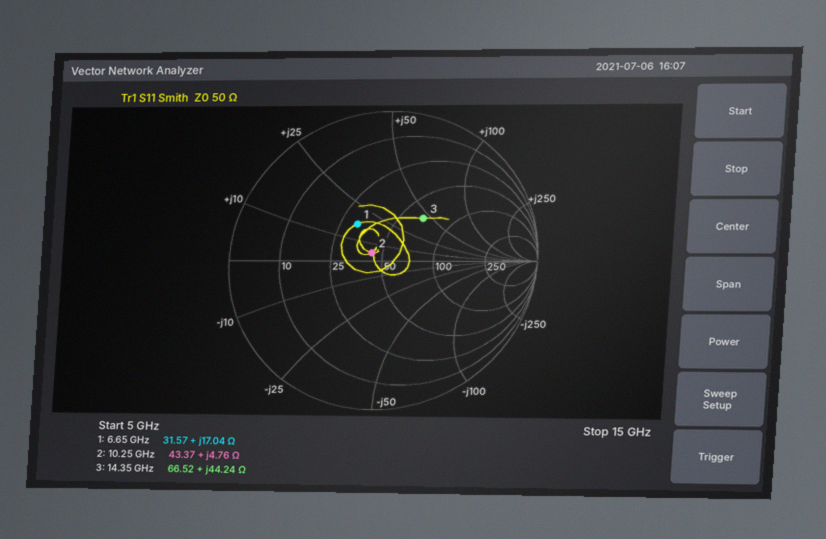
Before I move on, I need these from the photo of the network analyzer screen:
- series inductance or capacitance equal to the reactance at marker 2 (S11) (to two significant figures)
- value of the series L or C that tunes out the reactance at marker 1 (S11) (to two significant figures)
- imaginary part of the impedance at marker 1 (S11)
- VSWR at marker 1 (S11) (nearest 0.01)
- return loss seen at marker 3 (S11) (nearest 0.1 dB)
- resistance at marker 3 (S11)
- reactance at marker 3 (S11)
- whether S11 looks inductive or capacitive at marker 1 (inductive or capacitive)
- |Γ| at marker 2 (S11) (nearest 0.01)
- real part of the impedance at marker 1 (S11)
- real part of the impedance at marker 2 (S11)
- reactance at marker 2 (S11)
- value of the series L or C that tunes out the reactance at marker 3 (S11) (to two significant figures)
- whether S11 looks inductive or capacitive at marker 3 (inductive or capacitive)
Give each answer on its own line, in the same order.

74 pH
1.4 pF
+17.04 Ω
1.86
8.4 dB
66.52 Ω
+44.24 Ω
inductive
0.09
31.57 Ω
43.37 Ω
+4.76 Ω
250 fF
inductive
